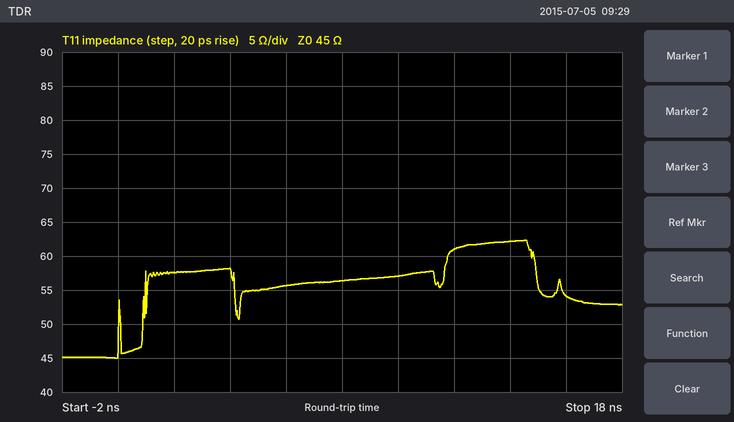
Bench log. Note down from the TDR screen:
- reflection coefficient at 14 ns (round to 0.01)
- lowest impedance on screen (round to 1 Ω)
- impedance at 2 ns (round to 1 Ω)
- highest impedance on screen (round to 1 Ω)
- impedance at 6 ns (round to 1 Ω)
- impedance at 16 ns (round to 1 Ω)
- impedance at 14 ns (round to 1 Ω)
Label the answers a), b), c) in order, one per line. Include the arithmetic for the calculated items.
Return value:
a) (62 − 45)/(62 + 45) ≈ +0.16
b) 45 Ω
c) 58 Ω
d) 62 Ω
e) 56 Ω
f) 54 Ω
g) 62 Ω
